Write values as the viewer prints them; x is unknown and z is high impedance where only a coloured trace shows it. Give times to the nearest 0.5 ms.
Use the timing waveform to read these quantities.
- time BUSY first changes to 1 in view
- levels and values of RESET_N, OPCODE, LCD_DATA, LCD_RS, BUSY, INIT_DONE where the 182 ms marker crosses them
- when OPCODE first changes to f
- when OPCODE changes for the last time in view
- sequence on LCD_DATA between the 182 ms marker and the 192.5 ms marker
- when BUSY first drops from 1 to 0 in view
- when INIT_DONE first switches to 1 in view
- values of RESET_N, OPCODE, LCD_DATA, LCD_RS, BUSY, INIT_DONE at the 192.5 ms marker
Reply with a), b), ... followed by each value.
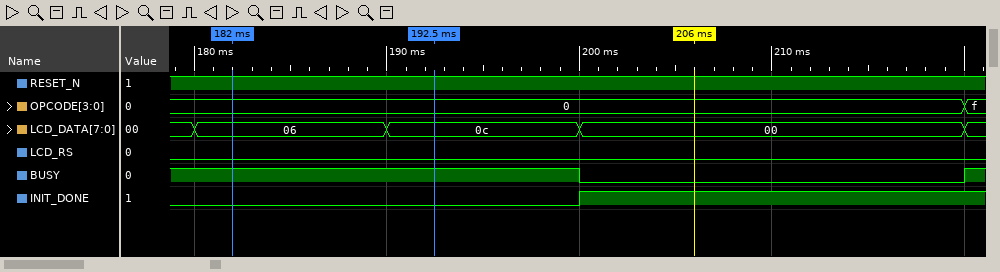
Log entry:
a) 220 ms
b) RESET_N=1, OPCODE=0, LCD_DATA=06, LCD_RS=0, BUSY=1, INIT_DONE=0
c) 220 ms
d) 220 ms
e) 06, 0c
f) 200 ms
g) 200 ms
h) RESET_N=1, OPCODE=0, LCD_DATA=0c, LCD_RS=0, BUSY=1, INIT_DONE=0
